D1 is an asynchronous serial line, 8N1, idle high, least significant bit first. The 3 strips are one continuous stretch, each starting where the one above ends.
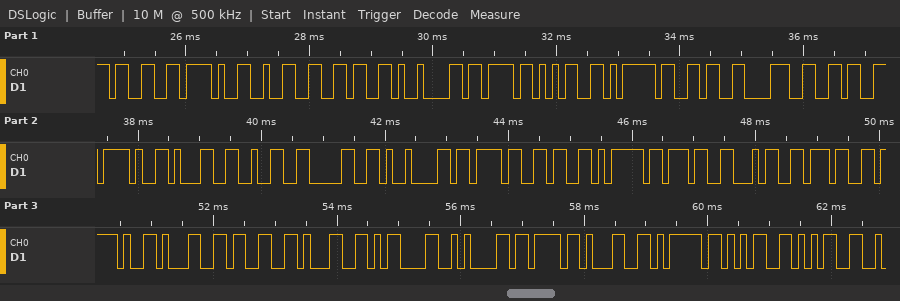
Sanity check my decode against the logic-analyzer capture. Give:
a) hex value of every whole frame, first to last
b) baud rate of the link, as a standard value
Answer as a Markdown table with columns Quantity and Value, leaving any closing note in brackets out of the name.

| Quantity | Value |
|---|---|
| hex value of every whole frame, first to last | 0x33 0x2F 0x32 0x36 0x09 0x7B 0x35 0x7D 0x36 0x38 0x36 0x2F 0x31 0x32 0x30 0x09 0x7B 0x36 0x7D 0x37 0x34 0x37 0x2F 0x31 0x33 0x31 0x0D 0x0A 0x7B 0x31 0x7D 0x35 0x35 |
| baud rate of the link, as a standard value | 9600 baud |
